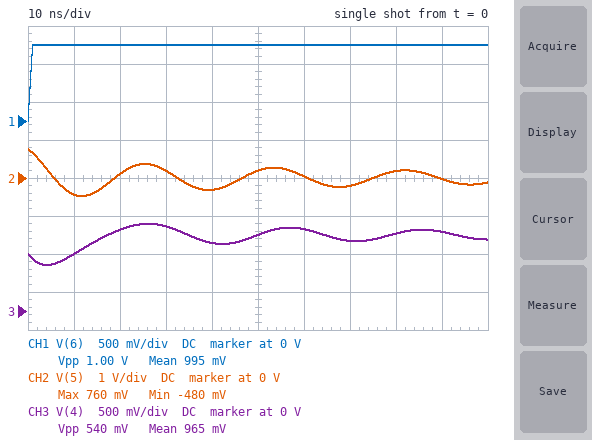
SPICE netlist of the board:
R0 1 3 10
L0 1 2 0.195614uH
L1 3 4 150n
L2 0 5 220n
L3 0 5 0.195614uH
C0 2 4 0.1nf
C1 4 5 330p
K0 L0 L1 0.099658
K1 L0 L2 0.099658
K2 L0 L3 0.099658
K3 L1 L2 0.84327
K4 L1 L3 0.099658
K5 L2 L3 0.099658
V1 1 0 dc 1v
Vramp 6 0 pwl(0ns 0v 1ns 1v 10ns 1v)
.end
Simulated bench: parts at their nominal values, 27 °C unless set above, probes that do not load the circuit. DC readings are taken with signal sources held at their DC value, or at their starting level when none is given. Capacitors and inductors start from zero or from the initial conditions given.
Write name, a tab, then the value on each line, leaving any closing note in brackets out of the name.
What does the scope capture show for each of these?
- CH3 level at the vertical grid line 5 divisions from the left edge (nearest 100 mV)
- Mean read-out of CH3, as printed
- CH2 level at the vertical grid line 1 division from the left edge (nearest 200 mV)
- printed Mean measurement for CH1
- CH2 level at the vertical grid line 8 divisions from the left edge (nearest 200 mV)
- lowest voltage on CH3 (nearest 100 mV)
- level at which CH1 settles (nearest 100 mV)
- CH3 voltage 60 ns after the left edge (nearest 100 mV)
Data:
CH3 level at the vertical grid line 5 divisions from the left edge	1.0 V
Mean read-out of CH3, as printed	965 mV
CH2 level at the vertical grid line 1 division from the left edge	-400 mV
printed Mean measurement for CH1	995 mV
CH2 level at the vertical grid line 8 divisions from the left edge	200 mV
lowest voltage on CH3	600 mV
level at which CH1 settles	1.0 V
CH3 voltage 60 ns after the left edge	1.1 V
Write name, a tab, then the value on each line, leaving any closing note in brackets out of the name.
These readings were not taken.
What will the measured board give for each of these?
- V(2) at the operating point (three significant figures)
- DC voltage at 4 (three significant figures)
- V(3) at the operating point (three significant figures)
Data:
V(2) at the operating point	1.00 V
DC voltage at 4	1.00 V
V(3) at the operating point	1.00 V
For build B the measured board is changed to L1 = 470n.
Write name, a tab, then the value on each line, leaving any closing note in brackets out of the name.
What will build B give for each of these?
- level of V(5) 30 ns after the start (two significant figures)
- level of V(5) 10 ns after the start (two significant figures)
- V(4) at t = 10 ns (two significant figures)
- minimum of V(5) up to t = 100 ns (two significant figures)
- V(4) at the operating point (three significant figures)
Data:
level of V(5) 30 ns after the start	280 mV
level of V(5) 10 ns after the start	-320 mV
V(4) at t = 10 ns	680 mV
minimum of V(5) up to t = 100 ns	-370 mV
V(4) at the operating point	1.00 V
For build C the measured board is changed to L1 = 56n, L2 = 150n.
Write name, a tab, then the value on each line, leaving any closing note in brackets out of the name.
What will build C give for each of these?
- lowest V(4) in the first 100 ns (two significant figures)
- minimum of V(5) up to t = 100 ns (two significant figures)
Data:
lowest V(4) in the first 100 ns	560 mV
minimum of V(5) up to t = 100 ns	-460 mV
